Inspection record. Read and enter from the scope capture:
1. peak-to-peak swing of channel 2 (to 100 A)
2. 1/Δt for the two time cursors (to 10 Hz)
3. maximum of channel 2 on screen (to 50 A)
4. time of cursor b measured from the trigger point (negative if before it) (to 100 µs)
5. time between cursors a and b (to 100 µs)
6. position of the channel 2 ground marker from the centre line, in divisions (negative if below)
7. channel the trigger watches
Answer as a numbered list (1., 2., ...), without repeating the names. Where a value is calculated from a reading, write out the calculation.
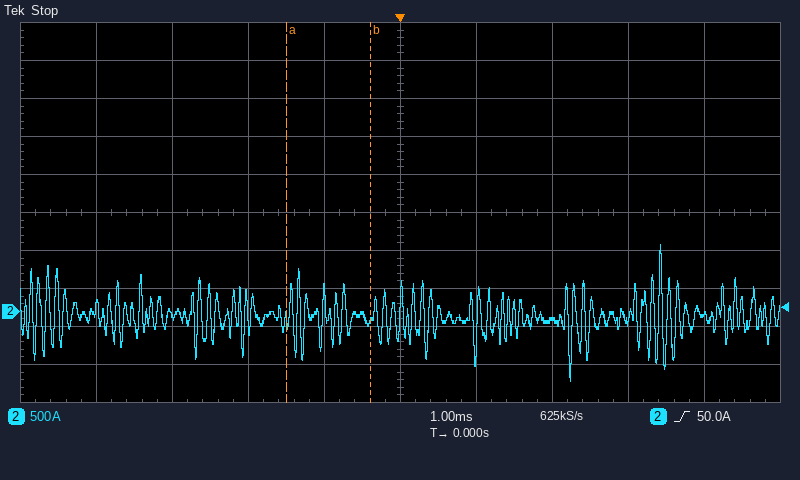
1. 1.80 kA
2. 1 / 1.1 ms ≈ 910 Hz
3. 900 A
4. -400 µs
5. 1.1 ms
6. -2.6 div
7. channel 2
